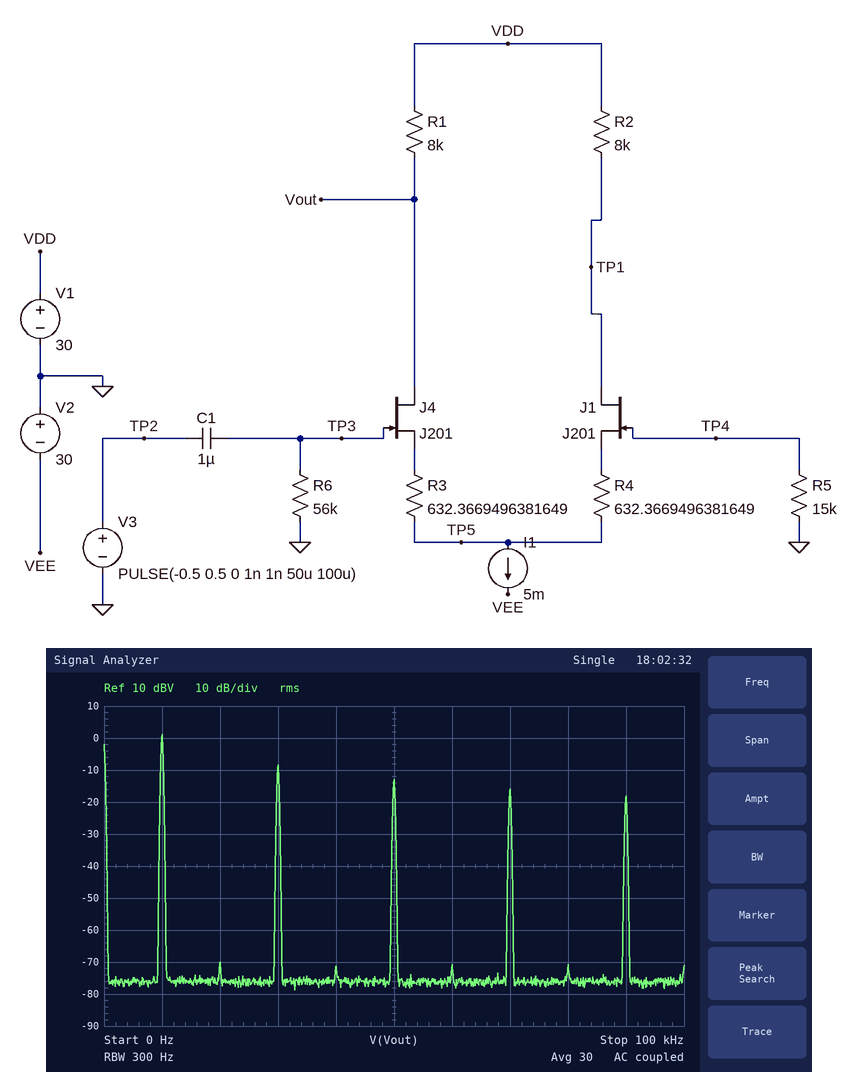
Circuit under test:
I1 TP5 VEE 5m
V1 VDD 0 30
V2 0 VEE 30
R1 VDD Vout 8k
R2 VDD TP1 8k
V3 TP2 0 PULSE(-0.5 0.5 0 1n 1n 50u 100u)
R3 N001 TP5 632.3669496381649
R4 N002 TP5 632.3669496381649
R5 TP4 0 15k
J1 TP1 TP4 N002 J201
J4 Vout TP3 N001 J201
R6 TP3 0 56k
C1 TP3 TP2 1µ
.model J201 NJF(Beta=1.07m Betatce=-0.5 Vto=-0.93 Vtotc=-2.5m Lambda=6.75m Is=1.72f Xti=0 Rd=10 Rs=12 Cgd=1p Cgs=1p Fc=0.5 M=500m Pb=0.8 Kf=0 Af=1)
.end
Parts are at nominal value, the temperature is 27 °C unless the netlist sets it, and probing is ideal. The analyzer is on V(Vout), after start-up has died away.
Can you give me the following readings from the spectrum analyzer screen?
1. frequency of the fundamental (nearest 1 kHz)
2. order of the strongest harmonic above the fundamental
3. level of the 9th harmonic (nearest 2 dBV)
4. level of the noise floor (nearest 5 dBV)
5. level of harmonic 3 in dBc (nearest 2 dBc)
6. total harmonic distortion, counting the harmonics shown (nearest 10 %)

10 kHz
3
-18 dBV
-75 dBV
-10 dBc
40 %
